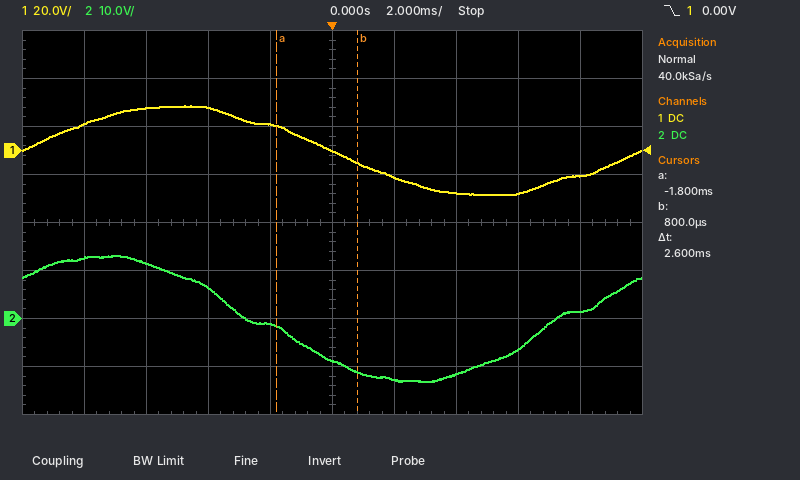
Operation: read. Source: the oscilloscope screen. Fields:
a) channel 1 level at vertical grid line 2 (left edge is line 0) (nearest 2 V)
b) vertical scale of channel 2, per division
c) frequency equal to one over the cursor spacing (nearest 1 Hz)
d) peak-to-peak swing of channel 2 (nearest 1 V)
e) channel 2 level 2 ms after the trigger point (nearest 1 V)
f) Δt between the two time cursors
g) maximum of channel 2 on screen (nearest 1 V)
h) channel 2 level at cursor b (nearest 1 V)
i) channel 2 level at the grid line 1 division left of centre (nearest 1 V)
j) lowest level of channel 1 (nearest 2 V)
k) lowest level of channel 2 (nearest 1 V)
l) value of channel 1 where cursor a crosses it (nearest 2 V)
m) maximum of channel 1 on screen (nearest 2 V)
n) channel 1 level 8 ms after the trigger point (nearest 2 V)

18 V
10 V
385 Hz
26 V
-13 V
2.6 ms
13 V
-11 V
-1 V
-18 V
-13 V
10 V
18 V
-10 V
